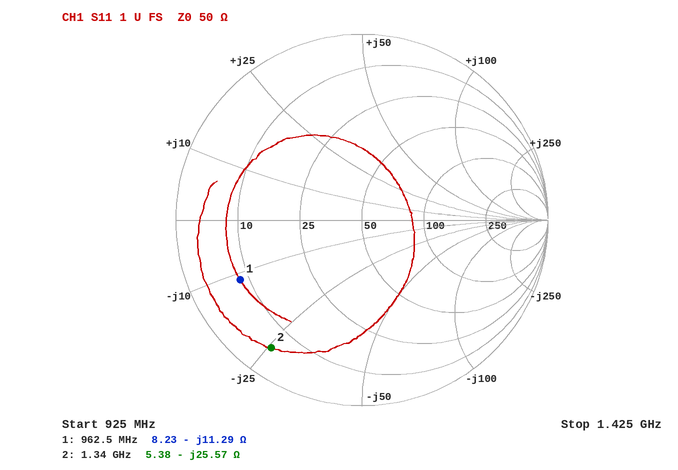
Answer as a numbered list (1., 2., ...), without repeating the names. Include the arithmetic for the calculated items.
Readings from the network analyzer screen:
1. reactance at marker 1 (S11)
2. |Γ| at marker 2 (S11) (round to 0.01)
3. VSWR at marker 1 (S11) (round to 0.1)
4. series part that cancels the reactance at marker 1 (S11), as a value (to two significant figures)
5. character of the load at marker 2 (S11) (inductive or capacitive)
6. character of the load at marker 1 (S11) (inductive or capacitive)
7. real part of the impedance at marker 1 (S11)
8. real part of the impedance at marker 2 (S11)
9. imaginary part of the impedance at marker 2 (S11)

1. -11.29 Ω
2. 0.84
3. 6.4
4. L = 11.29 Ω/(2π × 962.5 MHz) ≈ 1.9 nH
5. capacitive
6. capacitive
7. 8.23 Ω
8. 5.38 Ω
9. -25.57 Ω
